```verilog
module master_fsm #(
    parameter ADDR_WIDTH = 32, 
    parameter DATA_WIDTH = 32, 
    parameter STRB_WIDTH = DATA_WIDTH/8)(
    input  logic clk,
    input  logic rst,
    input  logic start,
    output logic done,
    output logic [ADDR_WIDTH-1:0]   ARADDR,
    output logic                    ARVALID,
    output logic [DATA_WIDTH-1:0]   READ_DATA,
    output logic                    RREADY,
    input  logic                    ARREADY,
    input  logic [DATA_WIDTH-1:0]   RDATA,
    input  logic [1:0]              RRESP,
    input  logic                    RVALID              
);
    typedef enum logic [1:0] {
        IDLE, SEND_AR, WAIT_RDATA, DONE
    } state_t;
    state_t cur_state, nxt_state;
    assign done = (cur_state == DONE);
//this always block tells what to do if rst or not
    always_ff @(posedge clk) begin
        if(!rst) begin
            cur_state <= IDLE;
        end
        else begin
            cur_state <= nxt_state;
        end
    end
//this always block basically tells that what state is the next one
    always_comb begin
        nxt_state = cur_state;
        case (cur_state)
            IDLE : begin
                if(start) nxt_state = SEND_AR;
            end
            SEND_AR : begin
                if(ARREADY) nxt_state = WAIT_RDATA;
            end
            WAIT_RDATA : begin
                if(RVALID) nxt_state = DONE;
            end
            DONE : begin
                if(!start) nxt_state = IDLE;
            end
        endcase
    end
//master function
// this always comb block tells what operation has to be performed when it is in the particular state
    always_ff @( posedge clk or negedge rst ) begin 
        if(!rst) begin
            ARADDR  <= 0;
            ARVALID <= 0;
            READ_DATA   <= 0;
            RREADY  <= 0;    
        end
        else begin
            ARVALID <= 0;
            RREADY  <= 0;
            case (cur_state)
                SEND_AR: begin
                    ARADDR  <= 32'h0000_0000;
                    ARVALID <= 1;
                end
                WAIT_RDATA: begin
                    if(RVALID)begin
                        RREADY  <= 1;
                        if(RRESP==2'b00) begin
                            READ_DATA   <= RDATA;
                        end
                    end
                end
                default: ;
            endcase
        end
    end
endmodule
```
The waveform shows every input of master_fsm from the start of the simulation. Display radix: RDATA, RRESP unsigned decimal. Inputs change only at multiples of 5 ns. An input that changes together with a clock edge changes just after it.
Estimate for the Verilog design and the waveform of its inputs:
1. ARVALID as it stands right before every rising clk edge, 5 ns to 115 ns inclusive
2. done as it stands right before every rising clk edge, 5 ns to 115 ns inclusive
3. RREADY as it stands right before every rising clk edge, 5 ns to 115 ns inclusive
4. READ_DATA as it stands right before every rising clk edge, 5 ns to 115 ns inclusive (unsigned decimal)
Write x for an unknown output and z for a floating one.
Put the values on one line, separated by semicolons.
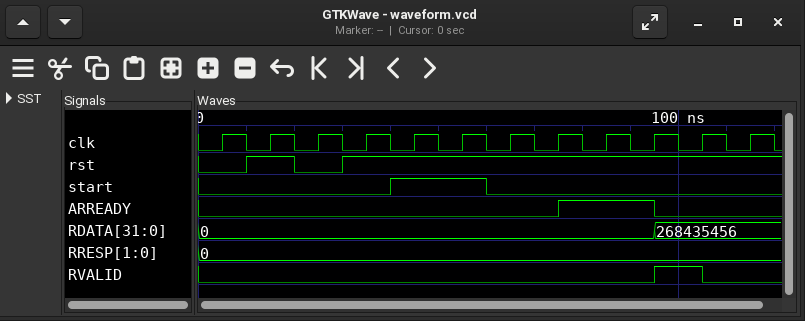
0 0 0 0 0 0 1 1 1 1 0 0; x 0 0 0 0 0 0 0 0 0 0 1; 0 0 0 0 0 0 0 0 0 0 0 1; 0, 0, 0, 0, 0, 0, 0, 0, 0, 0, 0, 268435456
